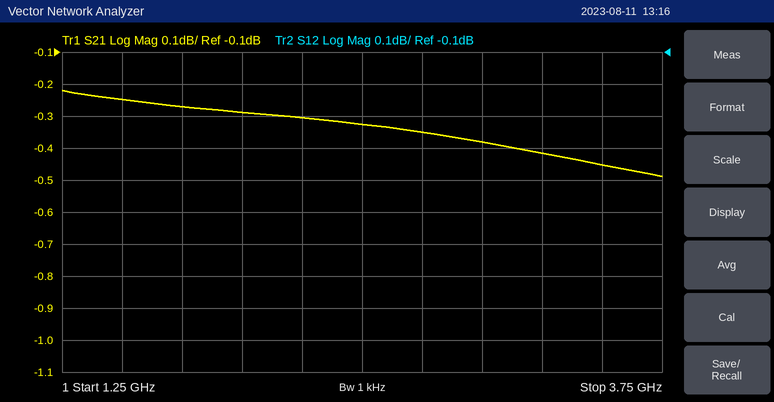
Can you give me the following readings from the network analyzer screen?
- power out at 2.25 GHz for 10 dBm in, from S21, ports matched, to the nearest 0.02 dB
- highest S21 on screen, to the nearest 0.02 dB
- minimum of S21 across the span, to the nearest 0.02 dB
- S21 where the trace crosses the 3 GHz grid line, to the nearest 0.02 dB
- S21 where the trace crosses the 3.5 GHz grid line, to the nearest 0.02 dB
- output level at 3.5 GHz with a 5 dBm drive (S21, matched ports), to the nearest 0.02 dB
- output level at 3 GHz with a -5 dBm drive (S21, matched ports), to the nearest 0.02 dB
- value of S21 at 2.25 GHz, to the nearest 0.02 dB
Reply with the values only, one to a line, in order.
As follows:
9.70 dBm
-0.22 dB
-0.48 dB
-0.38 dB
-0.46 dB
4.54 dBm
-5.38 dBm
-0.30 dB
